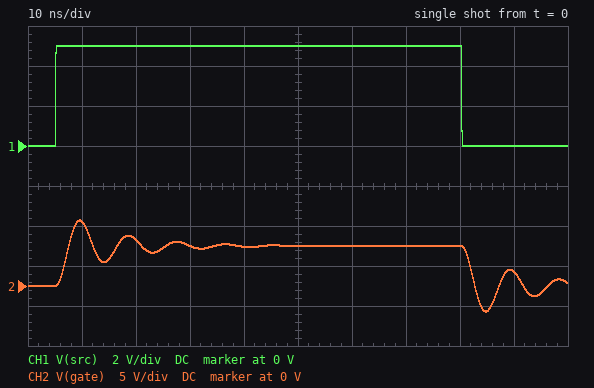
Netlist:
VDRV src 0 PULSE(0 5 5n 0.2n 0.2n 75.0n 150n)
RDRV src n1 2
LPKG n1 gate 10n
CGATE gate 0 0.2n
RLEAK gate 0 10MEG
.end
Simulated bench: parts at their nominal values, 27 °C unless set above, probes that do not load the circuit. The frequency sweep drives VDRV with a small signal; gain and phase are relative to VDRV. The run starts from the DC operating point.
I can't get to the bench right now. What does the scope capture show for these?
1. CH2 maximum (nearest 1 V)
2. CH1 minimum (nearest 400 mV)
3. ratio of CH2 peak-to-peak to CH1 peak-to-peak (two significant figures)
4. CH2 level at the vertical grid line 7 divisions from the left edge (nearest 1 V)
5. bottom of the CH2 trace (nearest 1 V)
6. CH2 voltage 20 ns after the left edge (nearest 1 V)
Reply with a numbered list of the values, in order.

1. 8 V
2. 0 V
3. 2.3
4. 5 V
5. -3 V
6. 6 V
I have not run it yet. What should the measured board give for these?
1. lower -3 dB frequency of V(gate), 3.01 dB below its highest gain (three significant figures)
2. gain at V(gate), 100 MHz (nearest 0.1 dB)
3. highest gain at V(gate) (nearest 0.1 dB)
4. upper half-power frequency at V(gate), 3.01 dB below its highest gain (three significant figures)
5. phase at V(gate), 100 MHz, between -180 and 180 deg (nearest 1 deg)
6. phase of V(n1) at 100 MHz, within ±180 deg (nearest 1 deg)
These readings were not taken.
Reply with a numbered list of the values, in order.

1. 92.8 MHz
2. 9.7 dB
3. 11.1 dB
4. 125 MHz
5. -50 deg
6. -50 deg
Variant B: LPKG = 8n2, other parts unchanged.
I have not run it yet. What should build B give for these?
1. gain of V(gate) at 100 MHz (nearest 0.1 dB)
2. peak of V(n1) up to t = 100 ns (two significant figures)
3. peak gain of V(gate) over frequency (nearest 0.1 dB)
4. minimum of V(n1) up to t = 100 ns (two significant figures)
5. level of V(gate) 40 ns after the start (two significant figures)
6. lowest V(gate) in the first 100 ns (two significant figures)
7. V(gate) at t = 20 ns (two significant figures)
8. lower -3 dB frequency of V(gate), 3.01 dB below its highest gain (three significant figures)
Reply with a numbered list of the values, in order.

1. 7.3 dB
2. 5.8 V
3. 10.2 dB
4. -760 mV
5. 5.0 V
6. -3.0 V
7. 4.7 V
8. 99.6 MHz
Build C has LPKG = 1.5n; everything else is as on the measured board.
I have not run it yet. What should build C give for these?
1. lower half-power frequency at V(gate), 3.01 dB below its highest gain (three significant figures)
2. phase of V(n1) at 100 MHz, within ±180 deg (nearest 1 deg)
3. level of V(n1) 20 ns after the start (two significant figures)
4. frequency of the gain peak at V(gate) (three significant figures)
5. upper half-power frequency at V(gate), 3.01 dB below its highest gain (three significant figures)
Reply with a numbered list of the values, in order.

1. 67.2 MHz
2. -16 deg
3. 5.0 V
4. 249 MHz
5. 345 MHz
